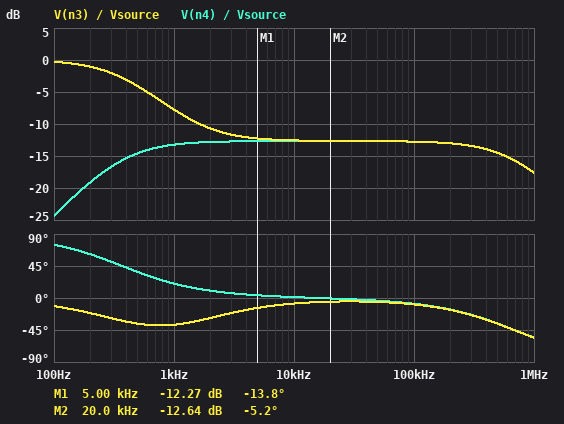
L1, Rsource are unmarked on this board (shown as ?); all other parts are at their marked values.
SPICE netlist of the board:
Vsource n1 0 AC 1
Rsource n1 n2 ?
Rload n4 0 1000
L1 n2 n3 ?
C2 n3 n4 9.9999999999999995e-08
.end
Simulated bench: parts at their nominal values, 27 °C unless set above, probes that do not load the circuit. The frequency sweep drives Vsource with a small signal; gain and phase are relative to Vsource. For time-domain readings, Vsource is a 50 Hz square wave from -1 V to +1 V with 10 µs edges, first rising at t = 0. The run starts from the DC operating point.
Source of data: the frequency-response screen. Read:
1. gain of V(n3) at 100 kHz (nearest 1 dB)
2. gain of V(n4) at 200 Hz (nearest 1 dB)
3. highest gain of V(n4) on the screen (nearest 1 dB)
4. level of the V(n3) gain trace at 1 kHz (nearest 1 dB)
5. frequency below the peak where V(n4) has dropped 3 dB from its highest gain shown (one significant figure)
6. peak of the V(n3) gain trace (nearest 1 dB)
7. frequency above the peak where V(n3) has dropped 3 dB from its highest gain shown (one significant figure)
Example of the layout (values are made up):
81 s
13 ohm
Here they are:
-13 dB
-19 dB
-13 dB
-8 dB
400 Hz
0 dB
400 Hz
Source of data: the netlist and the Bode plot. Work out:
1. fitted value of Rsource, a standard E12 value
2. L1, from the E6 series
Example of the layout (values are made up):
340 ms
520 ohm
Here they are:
3.3 kΩ
1 mH
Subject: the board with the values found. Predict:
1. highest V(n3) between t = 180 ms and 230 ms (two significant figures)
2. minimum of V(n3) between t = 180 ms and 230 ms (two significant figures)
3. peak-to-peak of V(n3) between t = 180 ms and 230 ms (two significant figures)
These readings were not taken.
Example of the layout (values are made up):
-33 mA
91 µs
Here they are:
1.0 V
-1.0 V
2.0 V
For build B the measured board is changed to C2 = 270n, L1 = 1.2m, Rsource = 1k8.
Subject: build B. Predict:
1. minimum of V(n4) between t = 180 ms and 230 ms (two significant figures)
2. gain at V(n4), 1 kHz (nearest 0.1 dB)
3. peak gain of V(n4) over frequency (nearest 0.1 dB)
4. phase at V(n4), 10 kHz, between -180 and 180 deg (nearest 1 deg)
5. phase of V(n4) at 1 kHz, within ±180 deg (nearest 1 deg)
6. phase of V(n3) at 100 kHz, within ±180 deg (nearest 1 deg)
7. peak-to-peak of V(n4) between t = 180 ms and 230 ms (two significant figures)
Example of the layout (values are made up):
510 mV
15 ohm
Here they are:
-710 mV
-9.1 dB
-8.9 dB
0 deg
12 deg
-15 deg
1.4 V
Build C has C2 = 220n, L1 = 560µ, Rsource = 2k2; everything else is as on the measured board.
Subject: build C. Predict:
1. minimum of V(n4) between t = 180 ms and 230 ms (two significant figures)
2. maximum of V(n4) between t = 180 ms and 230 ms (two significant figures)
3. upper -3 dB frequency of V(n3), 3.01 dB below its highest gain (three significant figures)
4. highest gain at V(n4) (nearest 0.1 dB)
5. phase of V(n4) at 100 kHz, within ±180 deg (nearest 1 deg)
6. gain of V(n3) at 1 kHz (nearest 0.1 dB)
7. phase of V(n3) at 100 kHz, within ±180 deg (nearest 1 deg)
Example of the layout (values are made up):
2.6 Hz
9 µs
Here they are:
-620 mV
620 mV
252 Hz
-10.1 dB
-6 deg
-8.5 dB
-7 deg
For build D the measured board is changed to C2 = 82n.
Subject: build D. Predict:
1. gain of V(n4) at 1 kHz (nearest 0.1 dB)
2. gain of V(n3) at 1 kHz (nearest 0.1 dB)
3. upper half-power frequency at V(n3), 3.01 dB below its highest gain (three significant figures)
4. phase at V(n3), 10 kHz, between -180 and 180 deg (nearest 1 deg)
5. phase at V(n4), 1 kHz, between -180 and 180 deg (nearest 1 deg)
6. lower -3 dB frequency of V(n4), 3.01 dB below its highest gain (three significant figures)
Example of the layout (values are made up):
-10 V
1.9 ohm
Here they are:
-13.5 dB
-6.7 dB
478 Hz
-9 deg
24 deg
451 Hz
